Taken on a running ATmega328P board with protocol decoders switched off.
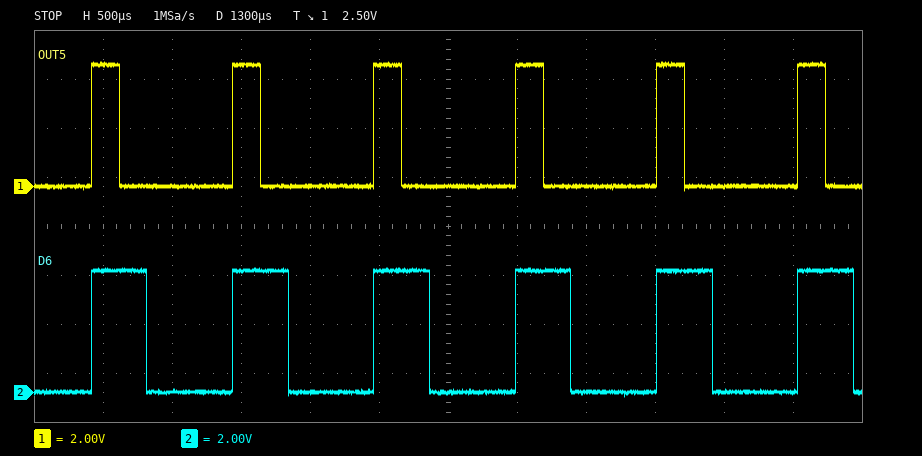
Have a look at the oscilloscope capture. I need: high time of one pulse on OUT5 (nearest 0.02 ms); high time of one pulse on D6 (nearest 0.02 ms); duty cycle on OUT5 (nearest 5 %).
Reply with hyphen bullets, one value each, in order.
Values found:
- 0.20 ms
- 0.40 ms
- 20 %
